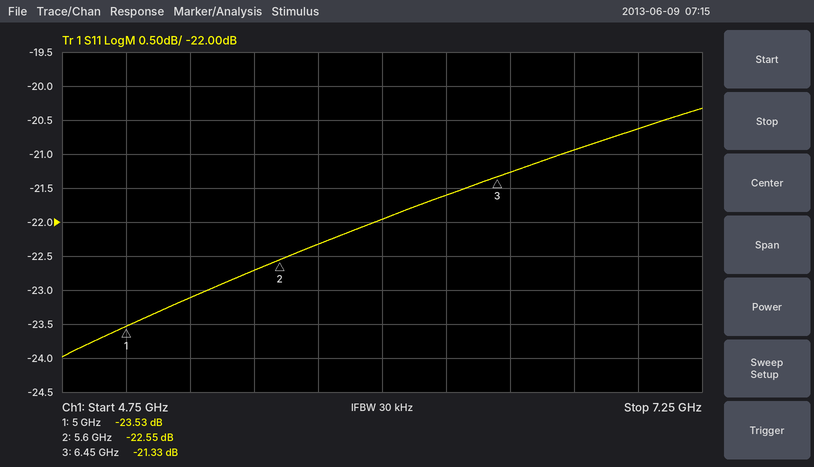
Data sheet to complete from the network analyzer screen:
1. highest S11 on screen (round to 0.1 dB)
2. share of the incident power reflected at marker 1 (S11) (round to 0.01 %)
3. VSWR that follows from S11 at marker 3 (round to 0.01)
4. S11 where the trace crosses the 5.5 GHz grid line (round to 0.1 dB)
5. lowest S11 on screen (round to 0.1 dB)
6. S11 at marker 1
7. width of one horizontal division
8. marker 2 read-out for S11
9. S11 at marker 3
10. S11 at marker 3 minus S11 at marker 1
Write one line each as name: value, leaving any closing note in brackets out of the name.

highest S11 on screen: -20.3 dB
share of the incident power reflected at marker 1 (S11): 0.44 %
VSWR that follows from S11 at marker 3: 1.19
S11 where the trace crosses the 5.5 GHz grid line: -22.7 dB
lowest S11 on screen: -24.0 dB
S11 at marker 1: -23.53 dB
width of one horizontal division: 250 MHz
marker 2 read-out for S11: -22.55 dB
S11 at marker 3: -21.33 dB
S11 at marker 3 minus S11 at marker 1: 2.20 dB
